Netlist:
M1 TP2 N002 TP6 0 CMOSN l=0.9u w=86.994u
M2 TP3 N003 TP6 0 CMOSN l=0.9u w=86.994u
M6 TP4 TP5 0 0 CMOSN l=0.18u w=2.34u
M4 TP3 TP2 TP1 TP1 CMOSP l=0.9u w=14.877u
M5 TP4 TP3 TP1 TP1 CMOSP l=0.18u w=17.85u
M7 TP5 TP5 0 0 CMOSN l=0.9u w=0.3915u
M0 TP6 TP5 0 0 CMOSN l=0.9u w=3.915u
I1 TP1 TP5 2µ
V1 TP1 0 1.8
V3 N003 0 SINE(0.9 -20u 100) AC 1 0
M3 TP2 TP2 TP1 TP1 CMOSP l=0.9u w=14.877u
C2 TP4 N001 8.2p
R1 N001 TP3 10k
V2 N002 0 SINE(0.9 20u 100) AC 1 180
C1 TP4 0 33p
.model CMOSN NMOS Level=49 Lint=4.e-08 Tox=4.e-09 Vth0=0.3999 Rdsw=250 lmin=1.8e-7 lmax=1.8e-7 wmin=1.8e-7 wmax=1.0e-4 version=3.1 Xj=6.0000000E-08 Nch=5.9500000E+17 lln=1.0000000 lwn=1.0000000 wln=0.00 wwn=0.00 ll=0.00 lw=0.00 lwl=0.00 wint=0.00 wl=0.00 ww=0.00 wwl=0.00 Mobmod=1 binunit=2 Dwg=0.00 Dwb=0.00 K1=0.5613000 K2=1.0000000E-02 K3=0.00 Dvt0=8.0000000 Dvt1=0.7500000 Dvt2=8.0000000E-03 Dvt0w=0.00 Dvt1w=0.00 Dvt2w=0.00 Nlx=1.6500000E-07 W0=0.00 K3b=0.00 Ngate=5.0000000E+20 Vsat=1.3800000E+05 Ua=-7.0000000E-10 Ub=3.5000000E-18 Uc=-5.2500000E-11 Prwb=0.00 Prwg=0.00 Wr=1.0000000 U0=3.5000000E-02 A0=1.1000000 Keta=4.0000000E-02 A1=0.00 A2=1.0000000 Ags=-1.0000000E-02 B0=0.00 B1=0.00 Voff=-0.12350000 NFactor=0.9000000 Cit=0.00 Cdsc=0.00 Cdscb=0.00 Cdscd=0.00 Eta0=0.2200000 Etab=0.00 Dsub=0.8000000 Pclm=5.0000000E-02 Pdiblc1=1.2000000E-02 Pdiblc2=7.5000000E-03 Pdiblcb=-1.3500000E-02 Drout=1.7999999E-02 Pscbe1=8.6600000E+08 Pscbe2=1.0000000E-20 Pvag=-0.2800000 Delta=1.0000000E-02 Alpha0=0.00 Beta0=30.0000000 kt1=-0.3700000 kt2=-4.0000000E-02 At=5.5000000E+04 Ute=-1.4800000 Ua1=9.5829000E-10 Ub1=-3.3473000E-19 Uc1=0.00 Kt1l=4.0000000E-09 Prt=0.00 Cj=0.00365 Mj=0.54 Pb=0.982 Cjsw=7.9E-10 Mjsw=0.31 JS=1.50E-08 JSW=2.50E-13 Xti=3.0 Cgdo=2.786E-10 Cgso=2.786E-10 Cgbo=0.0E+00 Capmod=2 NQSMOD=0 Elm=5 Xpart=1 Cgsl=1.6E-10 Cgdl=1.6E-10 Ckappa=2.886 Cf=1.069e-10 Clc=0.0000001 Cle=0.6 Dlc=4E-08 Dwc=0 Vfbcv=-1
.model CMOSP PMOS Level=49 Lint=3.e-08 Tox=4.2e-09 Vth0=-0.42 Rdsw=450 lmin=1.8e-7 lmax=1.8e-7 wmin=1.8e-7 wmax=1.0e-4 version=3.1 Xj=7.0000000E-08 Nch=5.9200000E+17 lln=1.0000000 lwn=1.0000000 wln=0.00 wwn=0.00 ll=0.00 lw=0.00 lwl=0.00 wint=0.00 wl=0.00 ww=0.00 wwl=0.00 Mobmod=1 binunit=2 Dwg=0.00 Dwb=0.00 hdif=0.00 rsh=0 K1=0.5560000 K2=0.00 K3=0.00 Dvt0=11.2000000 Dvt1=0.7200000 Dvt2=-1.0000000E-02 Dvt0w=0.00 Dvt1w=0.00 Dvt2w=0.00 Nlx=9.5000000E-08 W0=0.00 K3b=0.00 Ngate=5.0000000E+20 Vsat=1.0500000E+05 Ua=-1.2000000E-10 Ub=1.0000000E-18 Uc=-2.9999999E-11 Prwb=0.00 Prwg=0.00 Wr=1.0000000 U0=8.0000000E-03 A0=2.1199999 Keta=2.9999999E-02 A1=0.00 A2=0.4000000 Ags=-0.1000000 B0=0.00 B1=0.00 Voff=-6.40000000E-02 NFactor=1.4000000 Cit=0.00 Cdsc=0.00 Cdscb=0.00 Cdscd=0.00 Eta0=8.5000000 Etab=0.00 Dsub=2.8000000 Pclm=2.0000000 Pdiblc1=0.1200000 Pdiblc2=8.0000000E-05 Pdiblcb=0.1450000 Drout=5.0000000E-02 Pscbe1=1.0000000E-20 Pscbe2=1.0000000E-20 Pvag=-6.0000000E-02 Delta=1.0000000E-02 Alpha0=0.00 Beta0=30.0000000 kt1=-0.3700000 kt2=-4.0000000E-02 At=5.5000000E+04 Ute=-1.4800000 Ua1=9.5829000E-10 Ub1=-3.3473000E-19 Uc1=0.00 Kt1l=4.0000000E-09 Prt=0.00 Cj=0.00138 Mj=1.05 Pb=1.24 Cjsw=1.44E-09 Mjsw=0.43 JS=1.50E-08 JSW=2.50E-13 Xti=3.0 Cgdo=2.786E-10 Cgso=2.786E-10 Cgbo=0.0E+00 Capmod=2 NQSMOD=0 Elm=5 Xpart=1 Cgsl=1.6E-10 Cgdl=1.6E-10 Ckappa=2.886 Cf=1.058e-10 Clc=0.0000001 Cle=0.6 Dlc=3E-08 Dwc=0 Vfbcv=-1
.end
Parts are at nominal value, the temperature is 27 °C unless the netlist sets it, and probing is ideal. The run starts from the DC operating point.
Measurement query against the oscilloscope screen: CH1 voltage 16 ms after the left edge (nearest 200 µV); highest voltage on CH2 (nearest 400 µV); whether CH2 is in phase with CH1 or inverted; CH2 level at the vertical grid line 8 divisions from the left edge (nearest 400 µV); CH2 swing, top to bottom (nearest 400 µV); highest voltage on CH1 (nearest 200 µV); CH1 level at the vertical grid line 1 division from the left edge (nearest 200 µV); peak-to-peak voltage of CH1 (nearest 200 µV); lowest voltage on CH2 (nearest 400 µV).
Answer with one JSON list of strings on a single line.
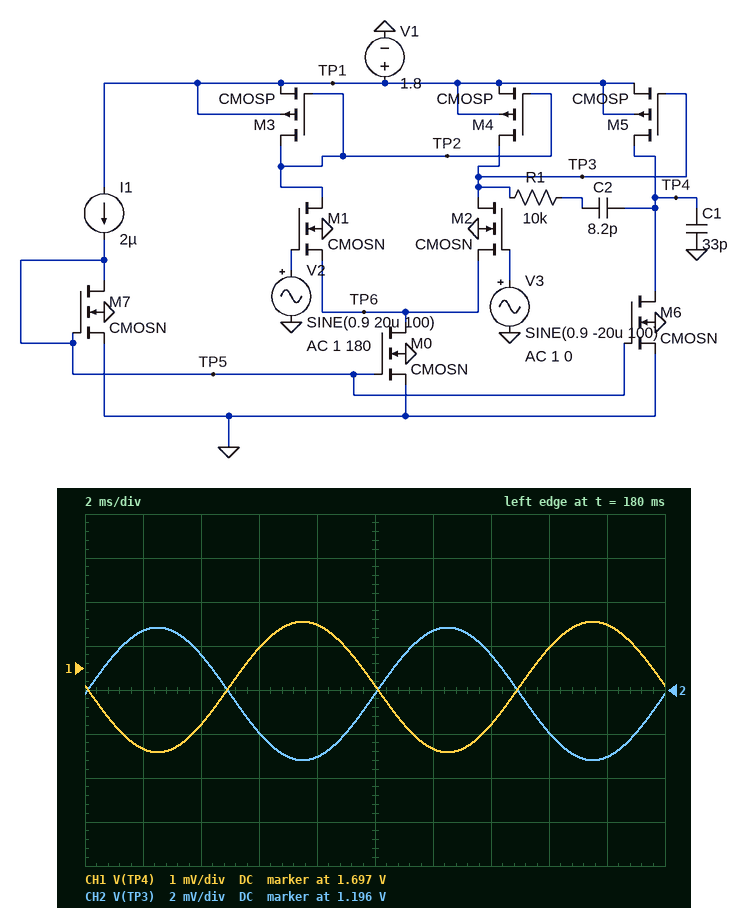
["1.6974 V", "1.1988 V", "inverted", "1.1940 V", "6.0 mV", "1.6980 V", "1.6952 V", "3.0 mV", "1.1928 V"]
